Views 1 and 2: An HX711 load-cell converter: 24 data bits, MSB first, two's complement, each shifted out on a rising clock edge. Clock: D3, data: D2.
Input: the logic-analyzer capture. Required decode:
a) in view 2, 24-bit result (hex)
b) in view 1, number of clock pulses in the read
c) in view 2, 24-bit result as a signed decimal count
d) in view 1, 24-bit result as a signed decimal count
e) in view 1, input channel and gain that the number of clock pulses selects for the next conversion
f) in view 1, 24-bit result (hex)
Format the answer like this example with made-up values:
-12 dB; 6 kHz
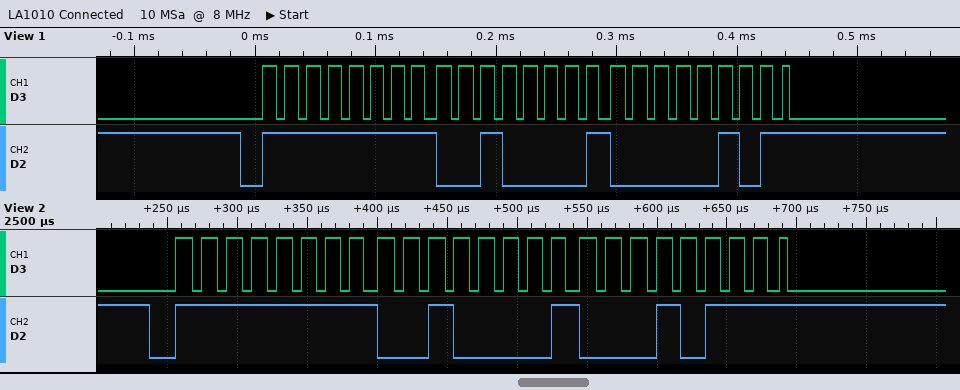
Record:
0xFF2117; 25; -57065; -57083; channel A, gain 128; 0xFF2105
